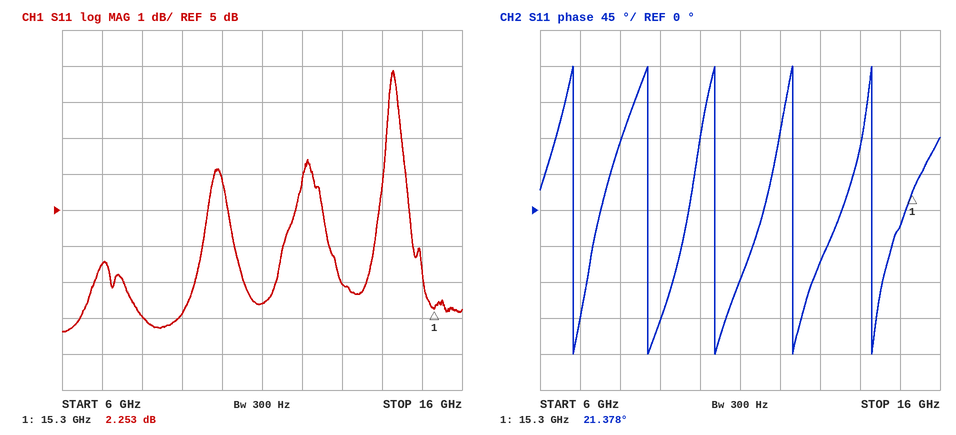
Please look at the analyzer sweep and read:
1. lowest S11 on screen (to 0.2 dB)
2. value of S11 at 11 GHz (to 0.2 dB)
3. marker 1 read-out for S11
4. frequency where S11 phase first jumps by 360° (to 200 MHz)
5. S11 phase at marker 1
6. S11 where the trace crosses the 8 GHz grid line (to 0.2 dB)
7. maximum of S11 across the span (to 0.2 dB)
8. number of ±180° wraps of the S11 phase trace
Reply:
1.6 dB
2.4 dB
2.253 dB
6.8 GHz
21.378°
2.0 dB
8.8 dB
5
